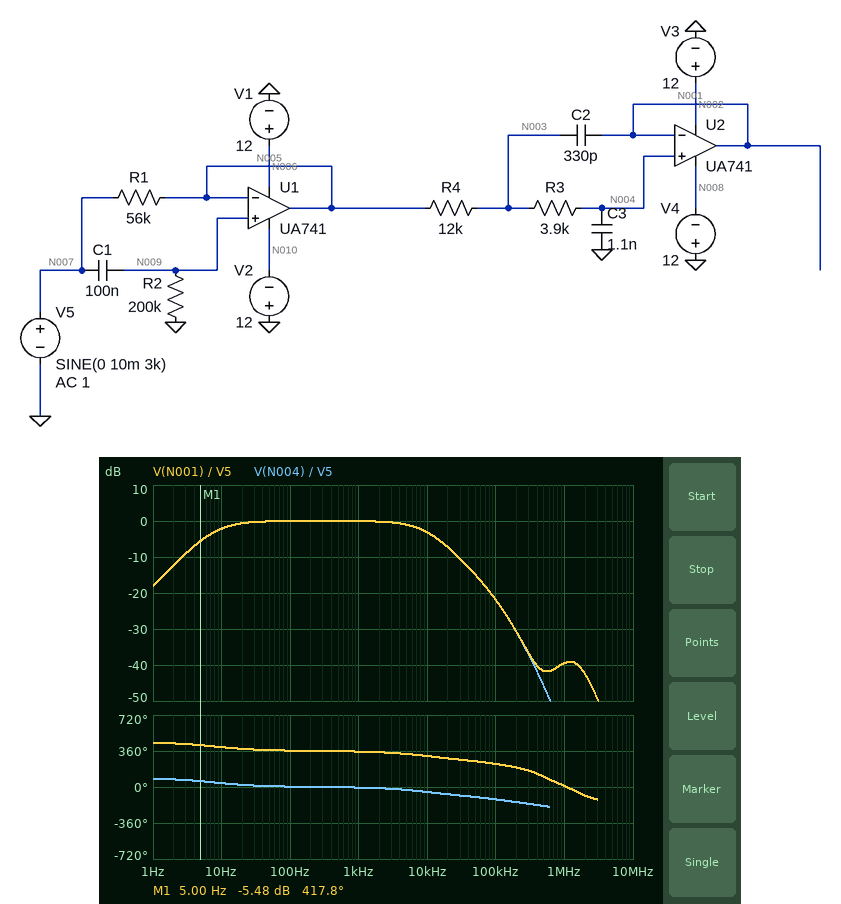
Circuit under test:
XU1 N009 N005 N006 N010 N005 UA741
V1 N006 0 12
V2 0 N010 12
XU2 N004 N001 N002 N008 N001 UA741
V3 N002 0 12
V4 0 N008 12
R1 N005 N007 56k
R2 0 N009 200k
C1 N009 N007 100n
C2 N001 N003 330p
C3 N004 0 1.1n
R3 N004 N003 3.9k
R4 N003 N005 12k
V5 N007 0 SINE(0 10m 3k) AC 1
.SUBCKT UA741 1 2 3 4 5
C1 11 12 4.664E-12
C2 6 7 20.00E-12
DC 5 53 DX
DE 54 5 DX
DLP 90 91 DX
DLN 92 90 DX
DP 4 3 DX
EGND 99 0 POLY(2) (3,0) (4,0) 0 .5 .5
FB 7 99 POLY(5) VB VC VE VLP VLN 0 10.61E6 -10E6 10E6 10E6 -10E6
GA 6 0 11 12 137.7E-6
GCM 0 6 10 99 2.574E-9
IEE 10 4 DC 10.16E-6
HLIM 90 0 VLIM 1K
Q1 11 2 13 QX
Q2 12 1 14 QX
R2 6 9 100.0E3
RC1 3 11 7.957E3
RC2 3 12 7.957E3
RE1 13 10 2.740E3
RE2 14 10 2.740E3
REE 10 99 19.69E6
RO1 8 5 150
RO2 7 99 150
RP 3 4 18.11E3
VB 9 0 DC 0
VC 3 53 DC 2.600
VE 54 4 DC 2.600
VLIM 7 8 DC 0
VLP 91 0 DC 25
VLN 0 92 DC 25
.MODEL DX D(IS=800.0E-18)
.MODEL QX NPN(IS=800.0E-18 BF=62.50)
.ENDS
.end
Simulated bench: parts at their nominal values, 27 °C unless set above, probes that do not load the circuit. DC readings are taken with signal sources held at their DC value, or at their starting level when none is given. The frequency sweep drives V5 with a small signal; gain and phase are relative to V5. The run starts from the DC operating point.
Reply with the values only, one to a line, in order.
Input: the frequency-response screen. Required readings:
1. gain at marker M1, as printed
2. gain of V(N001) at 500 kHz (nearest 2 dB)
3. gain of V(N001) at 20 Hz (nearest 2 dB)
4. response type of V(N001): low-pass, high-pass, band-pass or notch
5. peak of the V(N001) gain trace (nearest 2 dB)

-5.48 dB
-42 dB
0 dB
band-pass
0 dB
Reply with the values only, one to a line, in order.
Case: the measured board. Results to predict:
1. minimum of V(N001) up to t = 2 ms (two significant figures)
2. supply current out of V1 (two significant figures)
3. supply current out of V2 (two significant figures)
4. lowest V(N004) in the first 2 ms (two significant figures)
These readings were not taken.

-27 mV
1.3 mA
1.3 mA
-27 mV
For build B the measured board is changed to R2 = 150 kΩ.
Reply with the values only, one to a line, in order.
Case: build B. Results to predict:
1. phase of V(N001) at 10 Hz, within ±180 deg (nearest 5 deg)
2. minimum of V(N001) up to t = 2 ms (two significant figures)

45 deg
-23 mV
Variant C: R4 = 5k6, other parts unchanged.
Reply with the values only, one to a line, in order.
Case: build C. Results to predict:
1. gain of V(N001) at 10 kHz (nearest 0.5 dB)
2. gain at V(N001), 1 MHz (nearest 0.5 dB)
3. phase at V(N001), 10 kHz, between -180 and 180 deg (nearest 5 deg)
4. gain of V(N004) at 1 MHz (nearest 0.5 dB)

-1.5 dB
-33.0 dB
-35 deg
-53.5 dB
